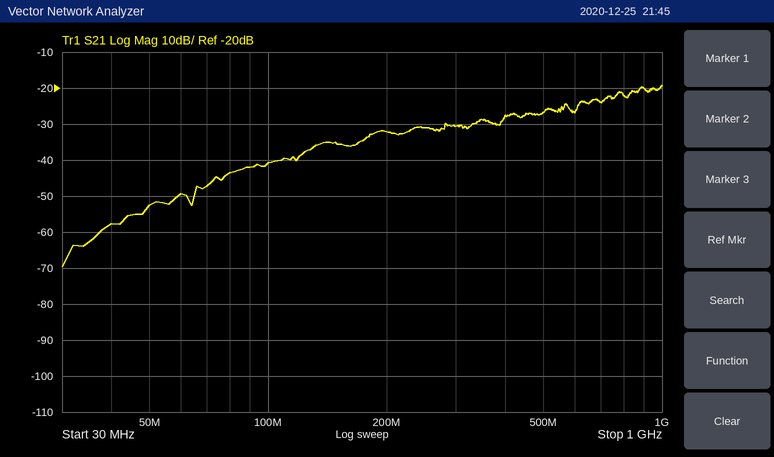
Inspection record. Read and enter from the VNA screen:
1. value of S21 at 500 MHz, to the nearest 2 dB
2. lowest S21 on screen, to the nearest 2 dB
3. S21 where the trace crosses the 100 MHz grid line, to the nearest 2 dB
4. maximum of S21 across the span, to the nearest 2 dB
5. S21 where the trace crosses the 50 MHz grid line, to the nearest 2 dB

-26 dB
-70 dB
-40 dB
-20 dB
-52 dB
